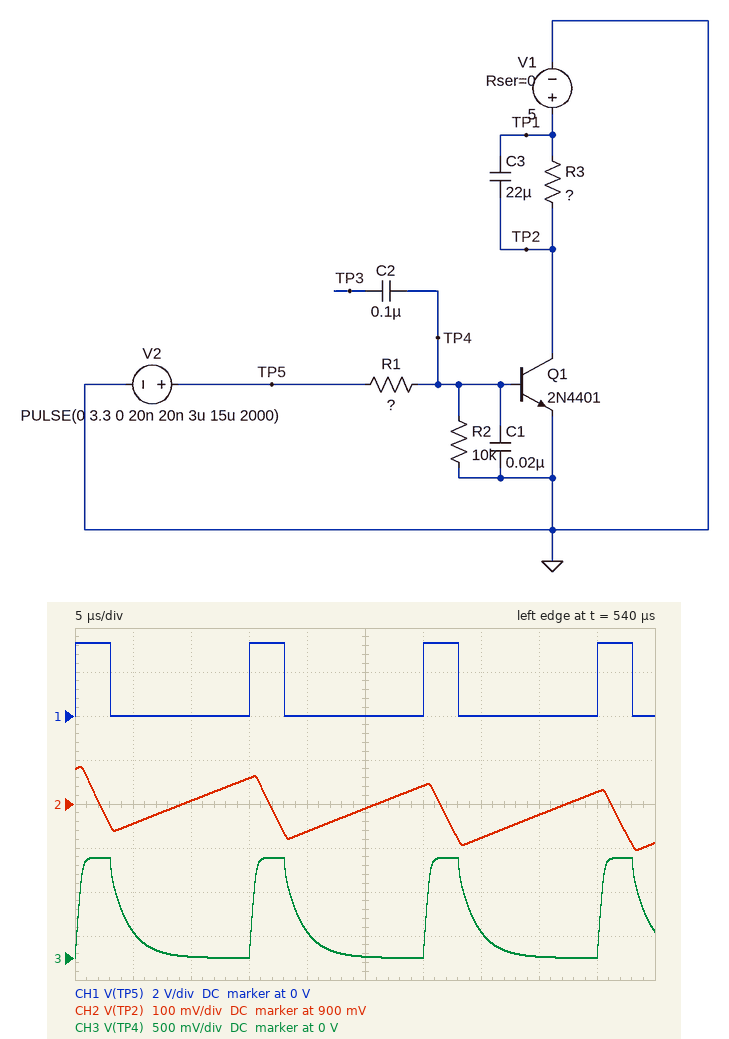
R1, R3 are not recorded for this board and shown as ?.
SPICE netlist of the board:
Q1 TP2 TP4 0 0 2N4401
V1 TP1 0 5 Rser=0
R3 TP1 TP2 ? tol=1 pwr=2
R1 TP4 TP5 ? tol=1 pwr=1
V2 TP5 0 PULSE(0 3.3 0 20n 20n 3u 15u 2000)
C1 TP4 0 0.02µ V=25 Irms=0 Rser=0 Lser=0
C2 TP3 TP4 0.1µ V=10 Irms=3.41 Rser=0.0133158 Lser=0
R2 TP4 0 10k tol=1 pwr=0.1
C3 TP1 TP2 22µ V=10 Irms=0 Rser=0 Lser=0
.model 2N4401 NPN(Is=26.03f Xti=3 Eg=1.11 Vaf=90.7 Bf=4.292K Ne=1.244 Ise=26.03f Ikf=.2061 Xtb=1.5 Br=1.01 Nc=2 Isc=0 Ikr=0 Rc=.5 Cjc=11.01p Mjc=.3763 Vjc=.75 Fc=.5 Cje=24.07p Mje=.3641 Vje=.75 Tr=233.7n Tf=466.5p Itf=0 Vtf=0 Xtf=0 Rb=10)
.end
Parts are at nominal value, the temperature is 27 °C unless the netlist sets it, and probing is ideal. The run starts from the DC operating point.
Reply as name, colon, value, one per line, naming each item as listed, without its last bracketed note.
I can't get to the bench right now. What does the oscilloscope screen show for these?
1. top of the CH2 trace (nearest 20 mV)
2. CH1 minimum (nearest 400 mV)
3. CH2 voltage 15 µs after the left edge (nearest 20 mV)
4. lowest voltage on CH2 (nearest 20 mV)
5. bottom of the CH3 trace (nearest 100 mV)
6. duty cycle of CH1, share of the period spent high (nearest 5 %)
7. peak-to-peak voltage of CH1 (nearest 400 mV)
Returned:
top of the CH2 trace: 980 mV
CH1 minimum: 0 V
CH2 voltage 15 µs after the left edge: 960 mV
lowest voltage on CH2: 800 mV
bottom of the CH3 trace: 0 V
duty cycle of CH1, share of the period spent high: 20 %
peak-to-peak voltage of CH1: 3.2 V
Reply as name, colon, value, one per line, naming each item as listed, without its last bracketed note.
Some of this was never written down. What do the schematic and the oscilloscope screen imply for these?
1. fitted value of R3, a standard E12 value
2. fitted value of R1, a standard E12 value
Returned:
fitted value of R3, a standard E12 value: 18 Ω
fitted value of R1, a standard E12 value: 82 Ω
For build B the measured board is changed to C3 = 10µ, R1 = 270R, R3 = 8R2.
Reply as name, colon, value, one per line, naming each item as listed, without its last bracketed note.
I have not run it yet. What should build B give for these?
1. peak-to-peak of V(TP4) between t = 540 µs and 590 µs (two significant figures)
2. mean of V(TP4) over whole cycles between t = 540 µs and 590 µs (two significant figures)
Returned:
peak-to-peak of V(TP4) between t = 540 µs and 590 µs: 850 mV
mean of V(TP4) over whole cycles between t = 540 µs and 590 µs: 410 mV
